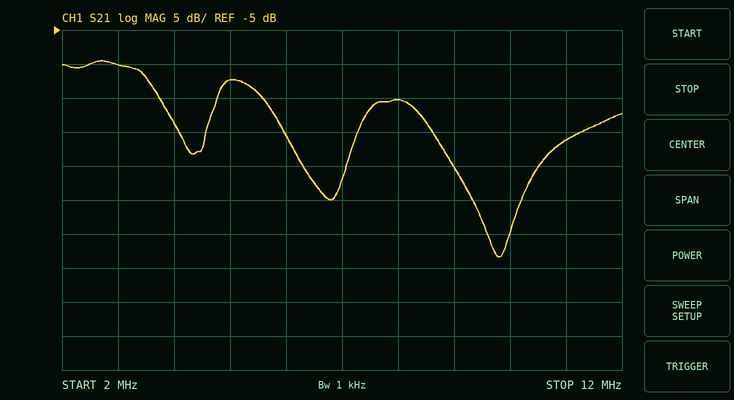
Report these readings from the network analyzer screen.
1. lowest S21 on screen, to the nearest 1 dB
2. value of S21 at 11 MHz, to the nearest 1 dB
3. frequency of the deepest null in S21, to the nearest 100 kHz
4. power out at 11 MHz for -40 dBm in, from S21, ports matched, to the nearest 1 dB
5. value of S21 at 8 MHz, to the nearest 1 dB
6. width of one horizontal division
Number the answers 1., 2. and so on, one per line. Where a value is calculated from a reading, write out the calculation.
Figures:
1. -38 dB
2. -21 dB
3. 9.8 MHz
4. -40 dBm + (-21 dB) = -61 dBm
5. -15 dB
6. 1 MHz
